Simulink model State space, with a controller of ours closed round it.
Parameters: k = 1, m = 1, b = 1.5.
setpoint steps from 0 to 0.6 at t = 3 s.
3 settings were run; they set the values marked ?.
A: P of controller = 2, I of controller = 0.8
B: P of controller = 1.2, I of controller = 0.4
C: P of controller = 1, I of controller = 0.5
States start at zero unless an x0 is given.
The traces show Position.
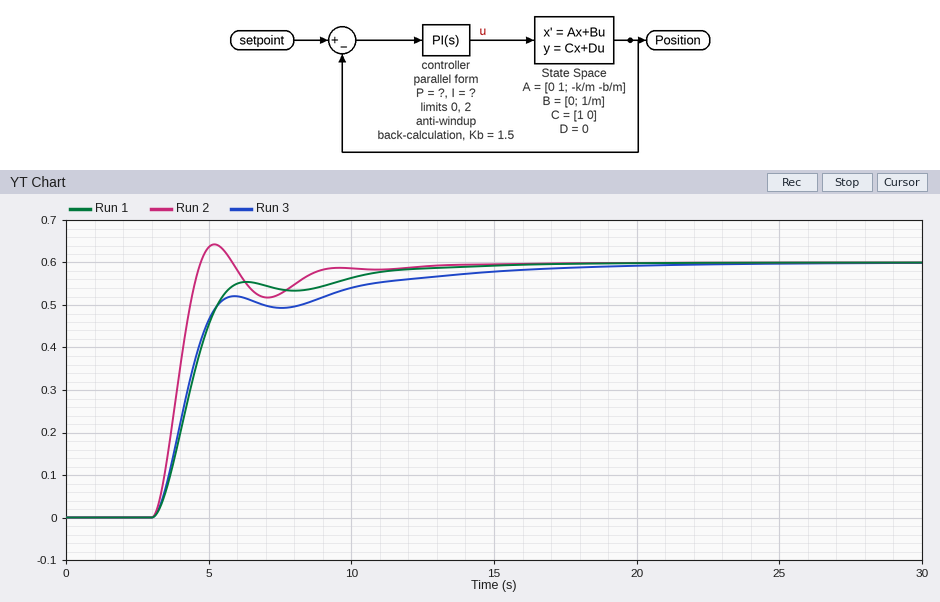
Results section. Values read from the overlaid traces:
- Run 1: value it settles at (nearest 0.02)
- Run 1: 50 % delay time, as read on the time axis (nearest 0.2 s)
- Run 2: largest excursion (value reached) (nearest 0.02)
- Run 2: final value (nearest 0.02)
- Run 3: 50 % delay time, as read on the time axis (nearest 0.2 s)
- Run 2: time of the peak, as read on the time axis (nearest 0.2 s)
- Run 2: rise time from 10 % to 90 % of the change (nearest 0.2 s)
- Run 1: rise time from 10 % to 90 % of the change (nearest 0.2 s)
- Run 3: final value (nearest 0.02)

0.60
4.4 s
0.64
0.60
4.2 s
5.2 s
1.2 s
2.2 s
0.60
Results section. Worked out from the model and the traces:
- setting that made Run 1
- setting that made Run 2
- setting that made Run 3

C
A
B
